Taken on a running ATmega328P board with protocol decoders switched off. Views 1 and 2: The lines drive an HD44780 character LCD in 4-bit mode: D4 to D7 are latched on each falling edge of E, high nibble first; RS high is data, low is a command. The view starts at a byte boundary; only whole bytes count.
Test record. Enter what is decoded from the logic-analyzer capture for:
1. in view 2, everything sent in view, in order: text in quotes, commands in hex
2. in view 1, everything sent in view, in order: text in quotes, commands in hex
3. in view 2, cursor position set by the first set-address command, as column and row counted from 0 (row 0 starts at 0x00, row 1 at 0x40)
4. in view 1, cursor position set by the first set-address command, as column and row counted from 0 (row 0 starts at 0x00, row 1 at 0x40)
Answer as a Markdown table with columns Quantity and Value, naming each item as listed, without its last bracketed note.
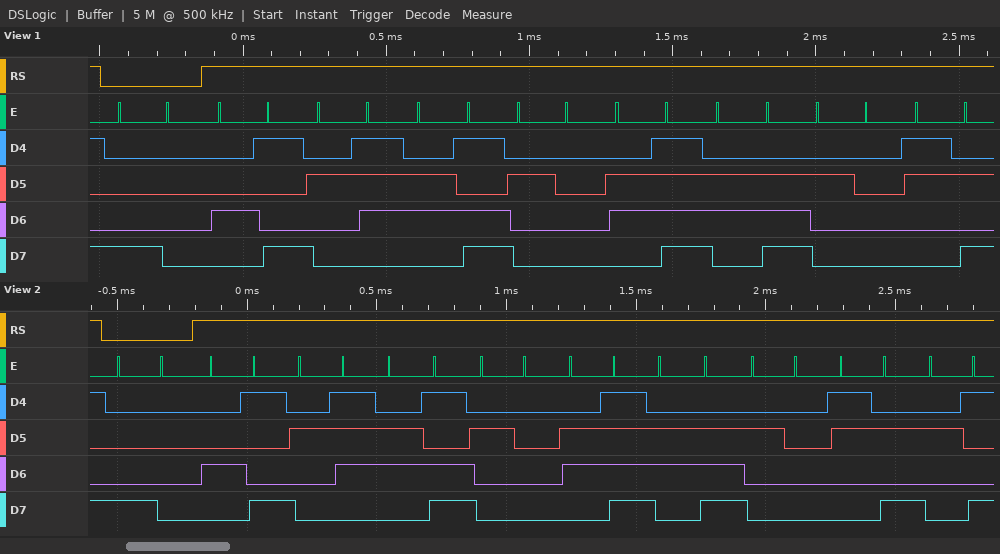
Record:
| Quantity | Value |
|---|---|
| in view 2, everything sent in view, in order: text in quotes, commands in hex | 0x80 "I'm on :)" |
| in view 1, everything sent in view, in order: text in quotes, commands in hex | 0x80 "I'm on :" |
| in view 2, cursor position set by the first set-address command, as column and row counted from 0 | column 0, row 0 |
| in view 1, cursor position set by the first set-address command, as column and row counted from 0 | column 0, row 0 |
